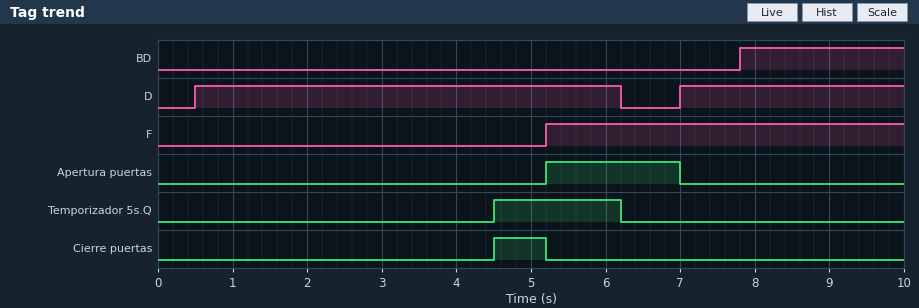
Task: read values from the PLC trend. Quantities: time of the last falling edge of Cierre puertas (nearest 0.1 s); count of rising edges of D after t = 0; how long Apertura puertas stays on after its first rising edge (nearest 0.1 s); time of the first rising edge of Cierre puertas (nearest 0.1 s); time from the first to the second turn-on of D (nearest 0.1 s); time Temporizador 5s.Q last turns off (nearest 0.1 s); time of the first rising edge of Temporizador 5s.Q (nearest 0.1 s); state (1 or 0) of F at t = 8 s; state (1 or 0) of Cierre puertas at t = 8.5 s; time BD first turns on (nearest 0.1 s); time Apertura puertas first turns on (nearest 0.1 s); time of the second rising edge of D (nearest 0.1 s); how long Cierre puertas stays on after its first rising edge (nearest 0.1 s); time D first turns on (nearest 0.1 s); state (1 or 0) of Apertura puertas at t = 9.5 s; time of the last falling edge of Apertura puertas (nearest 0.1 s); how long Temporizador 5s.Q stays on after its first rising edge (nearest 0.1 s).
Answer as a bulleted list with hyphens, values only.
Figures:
- 5.2 s
- 2
- 1.8 s
- 4.5 s
- 6.5 s
- 6.2 s
- 4.5 s
- 1
- 0
- 7.8 s
- 5.2 s
- 7.0 s
- 0.7 s
- 0.5 s
- 0
- 7.0 s
- 1.7 s
